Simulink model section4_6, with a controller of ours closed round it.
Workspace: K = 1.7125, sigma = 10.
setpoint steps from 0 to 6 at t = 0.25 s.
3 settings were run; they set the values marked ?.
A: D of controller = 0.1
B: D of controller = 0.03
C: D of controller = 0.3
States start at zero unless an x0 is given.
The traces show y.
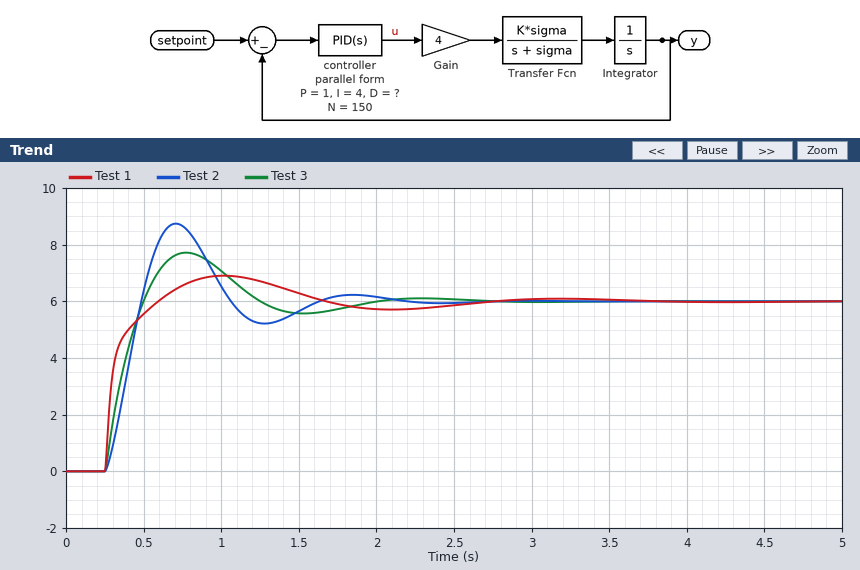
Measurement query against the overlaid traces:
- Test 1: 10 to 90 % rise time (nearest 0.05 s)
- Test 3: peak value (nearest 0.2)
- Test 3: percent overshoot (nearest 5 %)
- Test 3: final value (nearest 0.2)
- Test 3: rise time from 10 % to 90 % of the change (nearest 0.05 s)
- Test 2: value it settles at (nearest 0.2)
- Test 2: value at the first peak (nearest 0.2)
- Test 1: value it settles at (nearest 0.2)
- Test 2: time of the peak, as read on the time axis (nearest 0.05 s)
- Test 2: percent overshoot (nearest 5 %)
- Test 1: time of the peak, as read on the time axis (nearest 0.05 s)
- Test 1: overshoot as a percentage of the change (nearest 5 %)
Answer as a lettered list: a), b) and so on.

a) 0.20 s
b) 7.8
c) 30 %
d) 6.0
e) 0.20 s
f) 6.0
g) 8.8
h) 6.0
i) 0.70 s
j) 45 %
k) 1.00 s
l) 15 %
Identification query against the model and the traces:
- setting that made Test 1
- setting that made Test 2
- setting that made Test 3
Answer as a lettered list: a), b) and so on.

a) C
b) B
c) A
